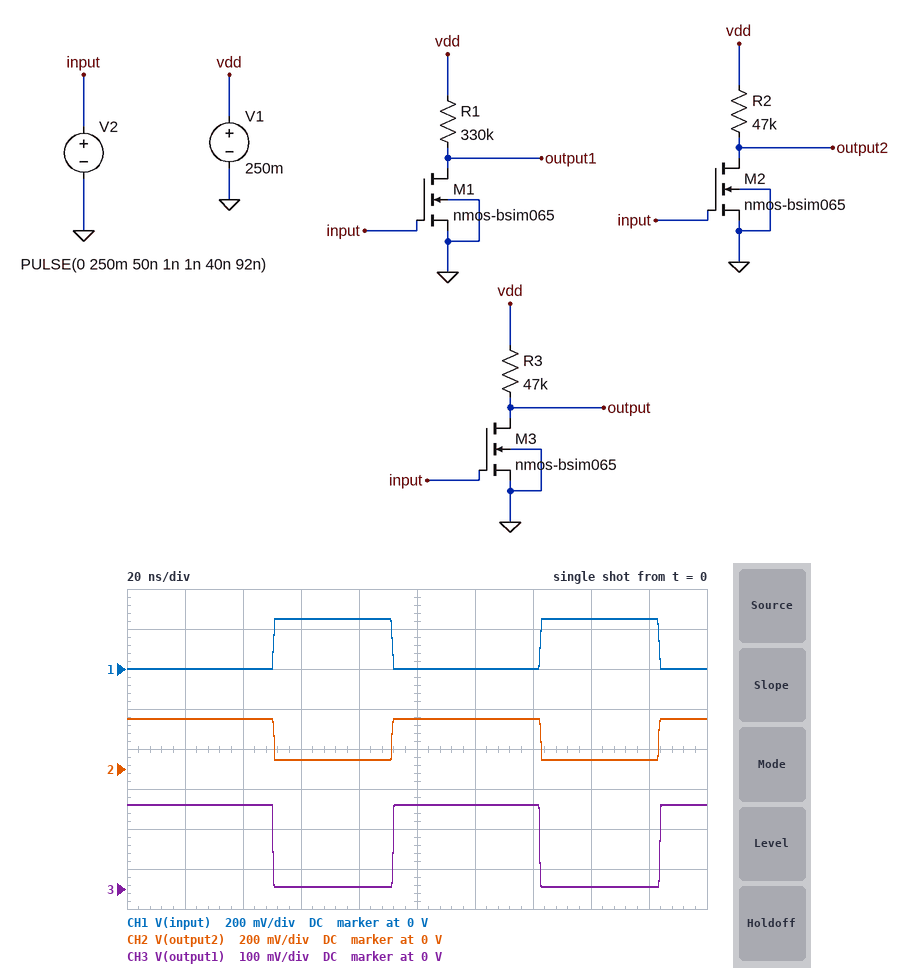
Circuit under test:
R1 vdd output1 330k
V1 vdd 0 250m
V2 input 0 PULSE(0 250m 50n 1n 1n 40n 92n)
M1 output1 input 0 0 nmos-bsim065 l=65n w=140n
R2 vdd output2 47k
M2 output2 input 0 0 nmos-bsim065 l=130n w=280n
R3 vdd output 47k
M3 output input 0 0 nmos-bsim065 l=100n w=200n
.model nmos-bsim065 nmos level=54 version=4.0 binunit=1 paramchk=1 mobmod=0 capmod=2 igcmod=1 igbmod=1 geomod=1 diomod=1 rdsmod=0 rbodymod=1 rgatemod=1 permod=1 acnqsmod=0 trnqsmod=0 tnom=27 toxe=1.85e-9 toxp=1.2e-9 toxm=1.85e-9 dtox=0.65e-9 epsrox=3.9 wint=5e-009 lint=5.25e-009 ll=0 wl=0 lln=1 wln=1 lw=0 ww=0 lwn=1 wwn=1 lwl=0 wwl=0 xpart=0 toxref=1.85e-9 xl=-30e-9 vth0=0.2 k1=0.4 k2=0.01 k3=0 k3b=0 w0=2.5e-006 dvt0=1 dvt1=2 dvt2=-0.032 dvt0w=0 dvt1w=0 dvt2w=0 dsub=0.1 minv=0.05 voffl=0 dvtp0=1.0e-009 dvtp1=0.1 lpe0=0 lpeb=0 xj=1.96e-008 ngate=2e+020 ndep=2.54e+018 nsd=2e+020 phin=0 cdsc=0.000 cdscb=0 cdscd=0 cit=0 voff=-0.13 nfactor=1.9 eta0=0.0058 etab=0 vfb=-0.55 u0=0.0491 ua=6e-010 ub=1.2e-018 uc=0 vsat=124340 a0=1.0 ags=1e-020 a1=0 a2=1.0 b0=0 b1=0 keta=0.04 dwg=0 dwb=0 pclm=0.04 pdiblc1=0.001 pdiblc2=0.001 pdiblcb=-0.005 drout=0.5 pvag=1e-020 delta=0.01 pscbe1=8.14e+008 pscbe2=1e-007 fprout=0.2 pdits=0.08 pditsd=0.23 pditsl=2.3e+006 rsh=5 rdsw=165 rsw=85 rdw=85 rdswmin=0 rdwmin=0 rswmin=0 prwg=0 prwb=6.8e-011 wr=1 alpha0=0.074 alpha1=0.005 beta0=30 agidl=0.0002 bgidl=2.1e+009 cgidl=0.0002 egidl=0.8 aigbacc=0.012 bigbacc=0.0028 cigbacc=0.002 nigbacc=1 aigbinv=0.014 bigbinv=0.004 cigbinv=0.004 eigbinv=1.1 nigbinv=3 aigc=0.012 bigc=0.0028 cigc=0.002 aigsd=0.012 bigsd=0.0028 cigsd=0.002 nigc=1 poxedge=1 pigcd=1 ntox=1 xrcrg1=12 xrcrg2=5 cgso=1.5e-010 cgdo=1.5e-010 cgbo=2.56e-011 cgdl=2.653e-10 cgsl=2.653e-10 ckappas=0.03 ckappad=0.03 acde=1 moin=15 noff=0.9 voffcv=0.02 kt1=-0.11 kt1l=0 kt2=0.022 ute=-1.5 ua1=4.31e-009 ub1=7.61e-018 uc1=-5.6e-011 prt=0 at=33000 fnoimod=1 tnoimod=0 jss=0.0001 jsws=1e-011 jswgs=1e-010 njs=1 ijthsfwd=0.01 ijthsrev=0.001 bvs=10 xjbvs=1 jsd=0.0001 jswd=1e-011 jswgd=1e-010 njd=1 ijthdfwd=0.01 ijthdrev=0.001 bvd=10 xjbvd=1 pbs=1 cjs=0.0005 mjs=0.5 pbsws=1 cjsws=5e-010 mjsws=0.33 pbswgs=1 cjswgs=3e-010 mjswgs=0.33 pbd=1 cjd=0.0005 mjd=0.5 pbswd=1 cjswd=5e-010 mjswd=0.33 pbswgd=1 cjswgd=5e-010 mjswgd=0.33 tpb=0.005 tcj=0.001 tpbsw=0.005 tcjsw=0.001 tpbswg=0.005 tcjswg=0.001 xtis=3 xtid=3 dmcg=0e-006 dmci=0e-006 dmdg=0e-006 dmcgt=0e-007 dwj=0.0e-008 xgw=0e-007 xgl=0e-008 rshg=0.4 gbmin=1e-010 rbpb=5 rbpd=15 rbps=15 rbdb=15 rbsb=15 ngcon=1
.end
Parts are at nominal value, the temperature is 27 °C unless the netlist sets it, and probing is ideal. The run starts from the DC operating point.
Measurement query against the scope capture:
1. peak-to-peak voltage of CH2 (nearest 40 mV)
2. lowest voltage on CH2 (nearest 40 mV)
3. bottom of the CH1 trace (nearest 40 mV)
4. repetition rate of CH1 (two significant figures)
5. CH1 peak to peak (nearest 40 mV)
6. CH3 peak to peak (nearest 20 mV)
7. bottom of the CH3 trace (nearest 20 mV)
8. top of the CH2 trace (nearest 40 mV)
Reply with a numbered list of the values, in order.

1. 200 mV
2. 40 mV
3. 0 V
4. 11 MHz
5. 240 mV
6. 200 mV
7. 0 V
8. 240 mV
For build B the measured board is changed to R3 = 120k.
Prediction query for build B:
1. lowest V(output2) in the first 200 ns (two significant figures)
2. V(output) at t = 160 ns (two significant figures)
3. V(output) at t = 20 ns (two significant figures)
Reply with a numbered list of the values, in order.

1. 43 mV
2. 16 mV
3. 240 mV
